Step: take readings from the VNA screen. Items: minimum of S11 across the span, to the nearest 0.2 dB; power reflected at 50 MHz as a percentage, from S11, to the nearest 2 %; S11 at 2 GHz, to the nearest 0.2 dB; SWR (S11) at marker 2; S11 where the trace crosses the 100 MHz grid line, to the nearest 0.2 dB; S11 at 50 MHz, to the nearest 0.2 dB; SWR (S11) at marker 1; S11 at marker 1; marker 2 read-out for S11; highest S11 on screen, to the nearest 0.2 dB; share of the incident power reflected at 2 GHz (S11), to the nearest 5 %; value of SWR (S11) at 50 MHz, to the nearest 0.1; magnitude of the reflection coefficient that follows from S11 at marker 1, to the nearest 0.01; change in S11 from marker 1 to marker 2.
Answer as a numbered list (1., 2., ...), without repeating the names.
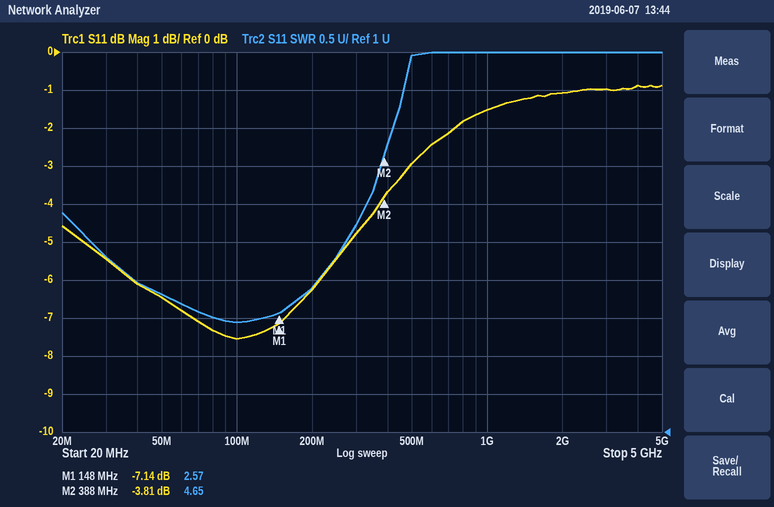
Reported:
1. -7.6 dB
2. 22 %
3. -1.0 dB
4. 4.65
5. -7.6 dB
6. -6.4 dB
7. 2.57
8. -7.14 dB
9. -3.81 dB
10. -0.8 dB
11. 80 %
12. 2.8
13. 0.44
14. 3.33 dB
